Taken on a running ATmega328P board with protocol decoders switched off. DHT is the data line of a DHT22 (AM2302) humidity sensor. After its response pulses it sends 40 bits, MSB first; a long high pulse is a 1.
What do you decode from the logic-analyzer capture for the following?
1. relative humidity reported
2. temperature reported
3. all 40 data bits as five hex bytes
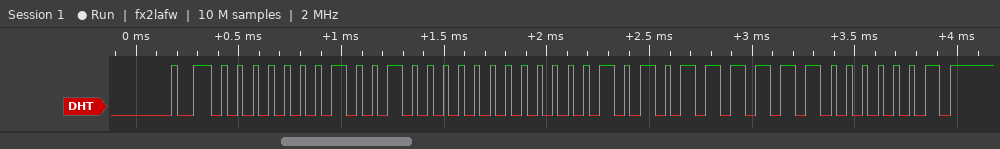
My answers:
28.8 %
35.1 °C
01 20 01 5F 81
